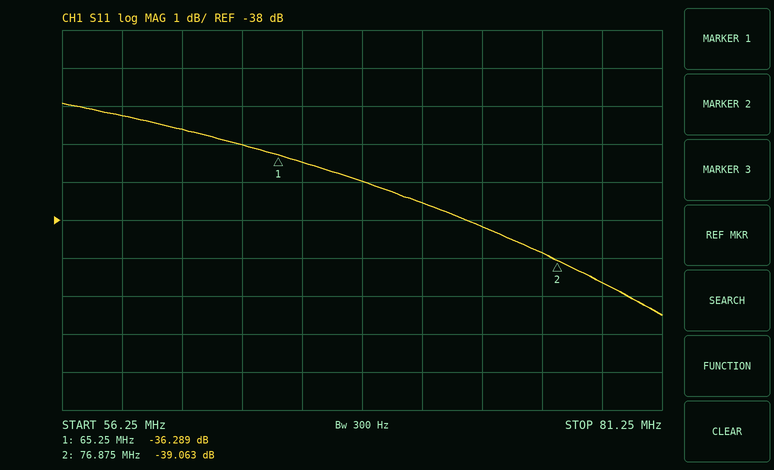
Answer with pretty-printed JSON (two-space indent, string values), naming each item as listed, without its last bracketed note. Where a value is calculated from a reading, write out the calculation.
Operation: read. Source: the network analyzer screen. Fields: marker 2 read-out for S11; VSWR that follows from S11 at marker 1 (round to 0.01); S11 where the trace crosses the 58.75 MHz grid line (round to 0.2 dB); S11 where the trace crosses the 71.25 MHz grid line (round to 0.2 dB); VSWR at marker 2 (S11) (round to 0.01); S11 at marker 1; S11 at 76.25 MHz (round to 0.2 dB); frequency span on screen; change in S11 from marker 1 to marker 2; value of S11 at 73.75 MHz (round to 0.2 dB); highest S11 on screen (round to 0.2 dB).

{
  "marker 2 read-out for S11": "-39.063 dB",
  "VSWR that follows from S11 at marker 1": "(1 + 0.0153)/(1 − 0.0153) ≈ 1.03",
  "S11 where the trace crosses the 58.75 MHz grid line": "-35.2 dB",
  "S11 where the trace crosses the 71.25 MHz grid line": "-37.6 dB",
  "VSWR at marker 2 (S11)": "(1 + 0.0111)/(1 − 0.0111) ≈ 1.02",
  "S11 at marker 1": "-36.289 dB",
  "S11 at 76.25 MHz": "-38.8 dB",
  "frequency span on screen": "25 MHz",
  "change in S11 from marker 1 to marker 2": "-39.063 − (-36.289) = -2.774 dB",
  "value of S11 at 73.75 MHz": "-38.2 dB",
  "highest S11 on screen": "-35.0 dB"
}
